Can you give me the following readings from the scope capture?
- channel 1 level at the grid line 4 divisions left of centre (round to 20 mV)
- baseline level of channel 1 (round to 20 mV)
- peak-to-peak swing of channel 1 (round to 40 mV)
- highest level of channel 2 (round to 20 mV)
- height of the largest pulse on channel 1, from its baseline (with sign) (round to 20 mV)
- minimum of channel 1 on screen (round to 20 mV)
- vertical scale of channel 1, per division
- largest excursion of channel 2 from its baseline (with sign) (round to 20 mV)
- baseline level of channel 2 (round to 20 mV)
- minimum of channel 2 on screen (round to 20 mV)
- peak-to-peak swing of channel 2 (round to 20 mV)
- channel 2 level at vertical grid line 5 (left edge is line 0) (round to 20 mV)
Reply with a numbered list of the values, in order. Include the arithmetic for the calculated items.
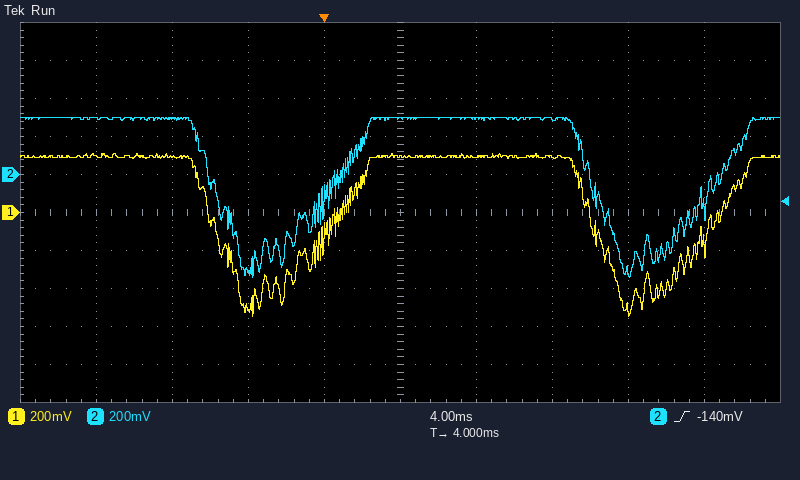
1. 300 mV
2. 300 mV
3. 840 mV
4. 300 mV
5. -540 mV − (300 mV) = -840 mV
6. -540 mV
7. 200 mV
8. -540 mV − (300 mV) = -840 mV
9. 300 mV
10. -540 mV
11. 300 mV − (-540 mV) = 840 mV
12. 300 mV
